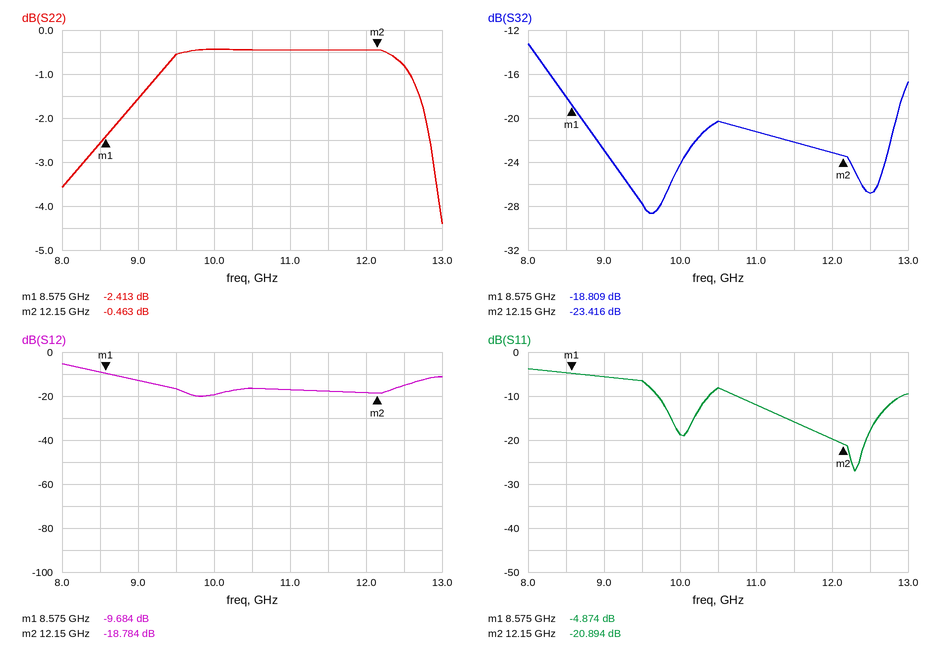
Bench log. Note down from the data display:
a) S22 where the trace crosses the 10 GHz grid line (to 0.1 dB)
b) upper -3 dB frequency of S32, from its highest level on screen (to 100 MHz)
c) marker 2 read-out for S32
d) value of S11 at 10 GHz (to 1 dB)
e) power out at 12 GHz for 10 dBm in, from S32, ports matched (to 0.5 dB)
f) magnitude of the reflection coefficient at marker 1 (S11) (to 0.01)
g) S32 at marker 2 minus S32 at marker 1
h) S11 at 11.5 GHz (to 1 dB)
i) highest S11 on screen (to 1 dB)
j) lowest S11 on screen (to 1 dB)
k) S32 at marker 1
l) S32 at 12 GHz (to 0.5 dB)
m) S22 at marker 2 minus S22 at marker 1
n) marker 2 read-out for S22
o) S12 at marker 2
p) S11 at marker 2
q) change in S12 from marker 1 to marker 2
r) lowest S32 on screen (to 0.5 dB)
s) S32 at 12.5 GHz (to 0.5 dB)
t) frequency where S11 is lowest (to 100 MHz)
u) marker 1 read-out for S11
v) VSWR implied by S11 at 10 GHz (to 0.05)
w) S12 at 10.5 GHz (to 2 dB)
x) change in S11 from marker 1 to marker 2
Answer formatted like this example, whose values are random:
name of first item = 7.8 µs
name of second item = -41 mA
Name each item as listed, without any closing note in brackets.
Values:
S22 where the trace crosses the 10 GHz grid line = -0.4 dB
upper -3 dB frequency of S32, from its highest level on screen = 8.3 GHz
marker 2 read-out for S32 = -23.416 dB
value of S11 at 10 GHz = -19 dB
power out at 12 GHz for 10 dBm in, from S32, ports matched = -13.0 dBm
magnitude of the reflection coefficient at marker 1 (S11) = 0.57
S32 at marker 2 minus S32 at marker 1 = -4.607 dB
S11 at 11.5 GHz = -16 dB
highest S11 on screen = -4 dB
lowest S11 on screen = -27 dB
S32 at marker 1 = -18.809 dB
S32 at 12 GHz = -23.0 dB
S22 at marker 2 minus S22 at marker 1 = 1.950 dB
marker 2 read-out for S22 = -0.463 dB
S12 at marker 2 = -18.784 dB
S11 at marker 2 = -20.894 dB
change in S12 from marker 1 to marker 2 = -9.100 dB
lowest S32 on screen = -28.5 dB
S32 at 12.5 GHz = -27.0 dB
frequency where S11 is lowest = 12.3 GHz
marker 1 read-out for S11 = -4.874 dB
VSWR implied by S11 at 10 GHz = 1.25
S12 at 10.5 GHz = -16 dB
change in S11 from marker 1 to marker 2 = -16.020 dB
